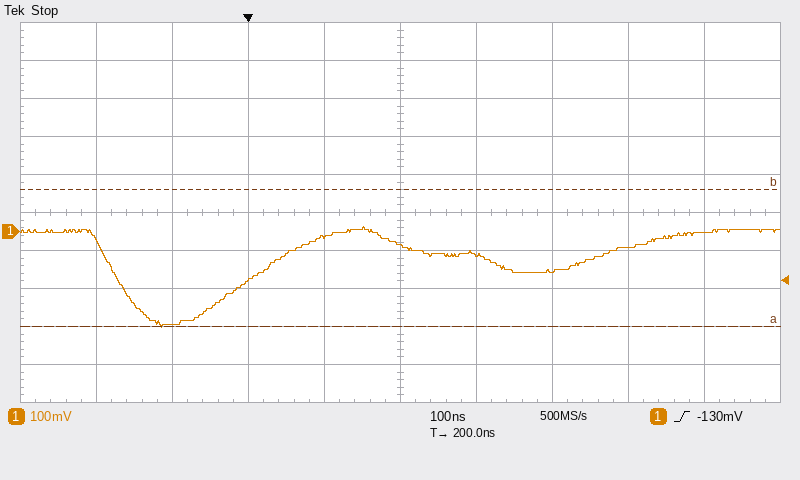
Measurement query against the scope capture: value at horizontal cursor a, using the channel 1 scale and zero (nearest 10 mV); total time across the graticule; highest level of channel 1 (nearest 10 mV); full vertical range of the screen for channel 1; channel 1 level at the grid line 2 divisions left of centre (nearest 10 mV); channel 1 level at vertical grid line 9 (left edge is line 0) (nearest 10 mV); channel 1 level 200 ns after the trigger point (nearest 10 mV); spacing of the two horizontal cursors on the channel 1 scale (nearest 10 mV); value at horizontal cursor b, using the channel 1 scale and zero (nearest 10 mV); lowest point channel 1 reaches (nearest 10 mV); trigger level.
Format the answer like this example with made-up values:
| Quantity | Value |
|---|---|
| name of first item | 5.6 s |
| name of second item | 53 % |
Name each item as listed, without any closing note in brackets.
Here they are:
| Quantity | Value |
|---|---|
| value at horizontal cursor a, using the channel 1 scale and zero | -250 mV |
| total time across the graticule | 1 µs |
| highest level of channel 1 | 10 mV |
| full vertical range of the screen for channel 1 | 1 V |
| channel 1 level at the grid line 2 divisions left of centre | -130 mV |
| channel 1 level at vertical grid line 9 (left edge is line 0) | 0 mV |
| channel 1 level 200 ns after the trigger point | -40 mV |
| spacing of the two horizontal cursors on the channel 1 scale | 360 mV |
| value at horizontal cursor b, using the channel 1 scale and zero | 110 mV |
| lowest point channel 1 reaches | -250 mV |
| trigger level | -130 mV |
